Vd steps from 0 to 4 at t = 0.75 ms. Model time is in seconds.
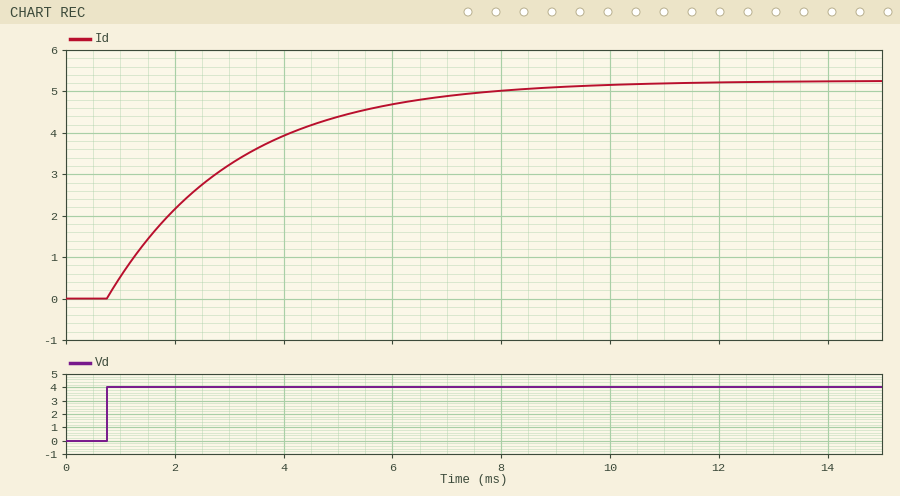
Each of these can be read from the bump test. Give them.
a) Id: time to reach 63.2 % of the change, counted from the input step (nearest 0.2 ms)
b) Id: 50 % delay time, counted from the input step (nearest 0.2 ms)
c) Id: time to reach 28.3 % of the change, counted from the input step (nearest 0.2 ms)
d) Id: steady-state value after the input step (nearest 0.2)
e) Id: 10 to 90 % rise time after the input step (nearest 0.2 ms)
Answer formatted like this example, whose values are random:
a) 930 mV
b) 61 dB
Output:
a) 2.4 ms
b) 1.6 ms
c) 0.8 ms
d) 5.2
e) 5.2 ms
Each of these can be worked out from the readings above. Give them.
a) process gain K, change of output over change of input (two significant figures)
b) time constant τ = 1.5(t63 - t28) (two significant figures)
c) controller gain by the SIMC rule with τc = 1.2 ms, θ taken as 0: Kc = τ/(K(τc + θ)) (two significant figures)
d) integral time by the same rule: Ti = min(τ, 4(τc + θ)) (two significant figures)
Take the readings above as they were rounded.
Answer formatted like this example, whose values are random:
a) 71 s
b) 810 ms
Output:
a) 1.3
b) 2.4 ms
c) 1.5
d) 2.4 ms
